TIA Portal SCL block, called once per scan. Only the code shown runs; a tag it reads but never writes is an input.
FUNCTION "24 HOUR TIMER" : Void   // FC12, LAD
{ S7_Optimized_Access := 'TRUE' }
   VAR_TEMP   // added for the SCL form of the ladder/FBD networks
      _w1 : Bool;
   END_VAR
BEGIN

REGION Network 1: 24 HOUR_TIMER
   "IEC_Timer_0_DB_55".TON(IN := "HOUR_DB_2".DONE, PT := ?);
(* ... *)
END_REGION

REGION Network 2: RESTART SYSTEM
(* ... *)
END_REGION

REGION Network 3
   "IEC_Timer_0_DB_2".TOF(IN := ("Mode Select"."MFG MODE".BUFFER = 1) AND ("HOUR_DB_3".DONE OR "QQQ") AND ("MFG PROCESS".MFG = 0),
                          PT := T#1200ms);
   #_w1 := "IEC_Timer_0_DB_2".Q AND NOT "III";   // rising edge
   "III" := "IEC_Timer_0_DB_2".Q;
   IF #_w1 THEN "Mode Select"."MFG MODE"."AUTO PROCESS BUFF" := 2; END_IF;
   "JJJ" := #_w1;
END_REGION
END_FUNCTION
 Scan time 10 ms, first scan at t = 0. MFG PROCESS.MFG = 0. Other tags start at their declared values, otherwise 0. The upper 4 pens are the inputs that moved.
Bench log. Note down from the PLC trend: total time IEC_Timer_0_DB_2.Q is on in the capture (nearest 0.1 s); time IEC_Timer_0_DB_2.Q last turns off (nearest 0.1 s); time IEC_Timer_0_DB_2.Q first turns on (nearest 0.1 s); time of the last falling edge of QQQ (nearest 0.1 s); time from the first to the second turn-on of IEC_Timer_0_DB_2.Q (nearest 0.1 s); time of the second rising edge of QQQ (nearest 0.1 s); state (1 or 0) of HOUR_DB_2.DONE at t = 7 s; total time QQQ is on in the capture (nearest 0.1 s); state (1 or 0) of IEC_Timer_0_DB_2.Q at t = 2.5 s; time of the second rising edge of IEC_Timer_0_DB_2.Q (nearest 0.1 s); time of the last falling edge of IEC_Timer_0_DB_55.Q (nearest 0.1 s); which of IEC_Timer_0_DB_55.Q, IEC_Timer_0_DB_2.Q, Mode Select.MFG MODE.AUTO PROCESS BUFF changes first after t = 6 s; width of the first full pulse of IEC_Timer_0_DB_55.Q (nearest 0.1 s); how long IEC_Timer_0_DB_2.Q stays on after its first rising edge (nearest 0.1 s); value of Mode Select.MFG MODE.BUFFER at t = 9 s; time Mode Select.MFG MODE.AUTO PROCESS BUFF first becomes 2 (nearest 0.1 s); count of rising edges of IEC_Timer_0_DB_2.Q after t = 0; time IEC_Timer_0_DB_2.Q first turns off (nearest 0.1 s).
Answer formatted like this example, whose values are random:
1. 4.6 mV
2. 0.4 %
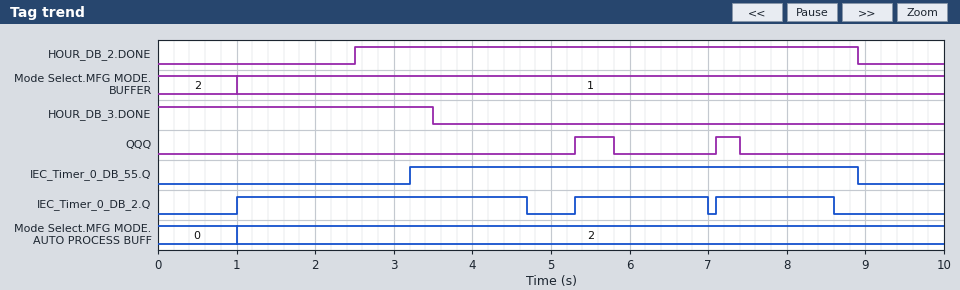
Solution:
1. 6.9 s
2. 8.6 s
3. 1.0 s
4. 7.4 s
5. 4.3 s
6. 7.1 s
7. 1
8. 0.8 s
9. 1
10. 5.3 s
11. 8.9 s
12. IEC_Timer_0_DB_2.Q
13. 5.7 s
14. 3.7 s
15. 1
16. 1.0 s
17. 3
18. 4.7 s
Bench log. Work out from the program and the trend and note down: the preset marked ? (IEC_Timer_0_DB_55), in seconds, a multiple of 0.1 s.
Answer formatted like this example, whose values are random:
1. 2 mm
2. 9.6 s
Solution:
1. 0.7 s
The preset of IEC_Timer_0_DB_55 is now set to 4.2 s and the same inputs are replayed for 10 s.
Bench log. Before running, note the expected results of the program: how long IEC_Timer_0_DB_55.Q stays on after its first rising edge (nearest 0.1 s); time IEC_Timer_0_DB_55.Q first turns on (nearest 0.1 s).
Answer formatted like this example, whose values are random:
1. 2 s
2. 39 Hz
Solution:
1. 2.2 s
2. 6.7 s
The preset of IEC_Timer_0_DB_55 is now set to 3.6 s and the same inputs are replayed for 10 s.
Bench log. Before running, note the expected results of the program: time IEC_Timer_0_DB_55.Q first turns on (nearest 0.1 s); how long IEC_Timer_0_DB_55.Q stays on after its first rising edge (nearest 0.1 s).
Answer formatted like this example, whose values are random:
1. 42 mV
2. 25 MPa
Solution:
1. 6.1 s
2. 2.8 s
